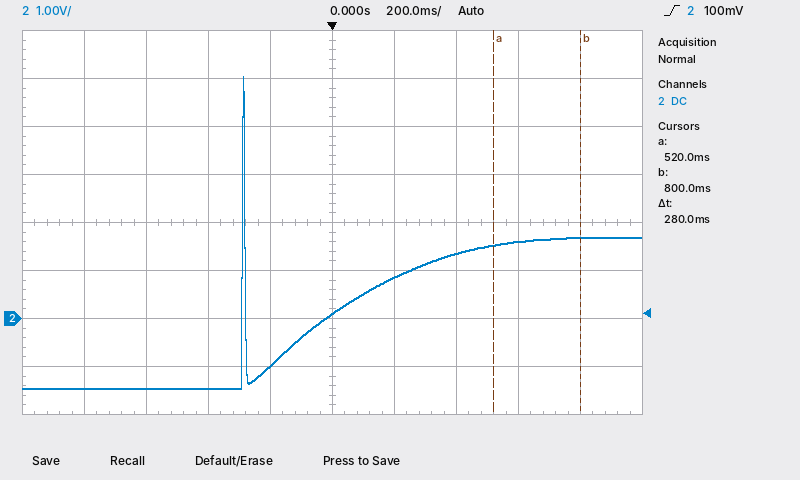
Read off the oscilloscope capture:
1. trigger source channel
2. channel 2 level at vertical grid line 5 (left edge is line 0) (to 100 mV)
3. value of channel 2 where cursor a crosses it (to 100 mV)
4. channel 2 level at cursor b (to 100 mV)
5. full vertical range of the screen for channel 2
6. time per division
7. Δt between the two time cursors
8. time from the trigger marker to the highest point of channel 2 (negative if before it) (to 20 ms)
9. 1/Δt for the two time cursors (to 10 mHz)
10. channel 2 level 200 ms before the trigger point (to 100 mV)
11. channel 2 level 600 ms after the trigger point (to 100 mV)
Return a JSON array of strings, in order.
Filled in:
["channel 2", "100 mV", "1.5 V", "1.7 V", "8 V", "200 ms", "280 ms", "-280 ms", "3.57 Hz", "-1.0 V", "1.6 V"]
